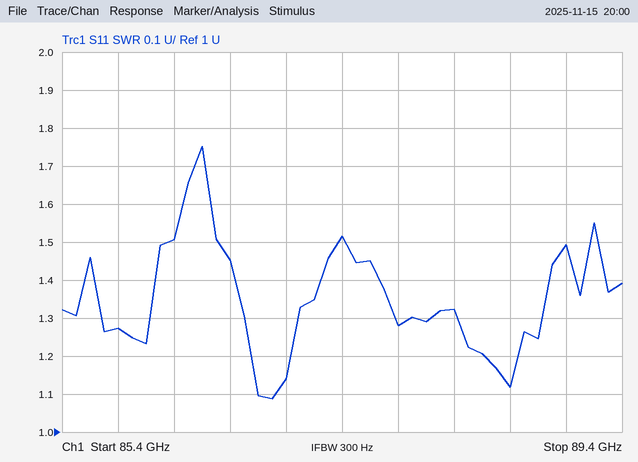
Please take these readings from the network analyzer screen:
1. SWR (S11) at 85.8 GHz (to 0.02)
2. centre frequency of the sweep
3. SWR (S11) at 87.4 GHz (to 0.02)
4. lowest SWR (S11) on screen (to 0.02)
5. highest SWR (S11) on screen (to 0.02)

1.28
87.4 GHz
1.52
1.08
1.76
